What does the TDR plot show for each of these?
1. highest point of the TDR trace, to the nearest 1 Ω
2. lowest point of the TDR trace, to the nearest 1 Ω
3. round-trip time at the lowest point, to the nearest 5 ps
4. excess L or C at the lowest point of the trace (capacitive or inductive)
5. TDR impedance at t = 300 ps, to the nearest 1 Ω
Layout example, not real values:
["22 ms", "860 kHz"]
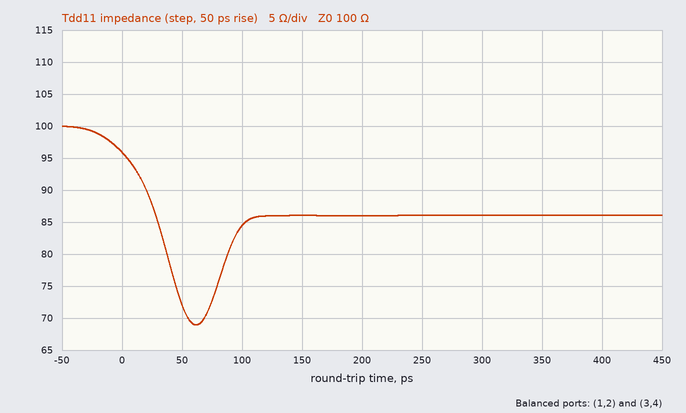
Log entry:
["100 Ω", "69 Ω", "60 ps", "capacitive", "86 Ω"]
